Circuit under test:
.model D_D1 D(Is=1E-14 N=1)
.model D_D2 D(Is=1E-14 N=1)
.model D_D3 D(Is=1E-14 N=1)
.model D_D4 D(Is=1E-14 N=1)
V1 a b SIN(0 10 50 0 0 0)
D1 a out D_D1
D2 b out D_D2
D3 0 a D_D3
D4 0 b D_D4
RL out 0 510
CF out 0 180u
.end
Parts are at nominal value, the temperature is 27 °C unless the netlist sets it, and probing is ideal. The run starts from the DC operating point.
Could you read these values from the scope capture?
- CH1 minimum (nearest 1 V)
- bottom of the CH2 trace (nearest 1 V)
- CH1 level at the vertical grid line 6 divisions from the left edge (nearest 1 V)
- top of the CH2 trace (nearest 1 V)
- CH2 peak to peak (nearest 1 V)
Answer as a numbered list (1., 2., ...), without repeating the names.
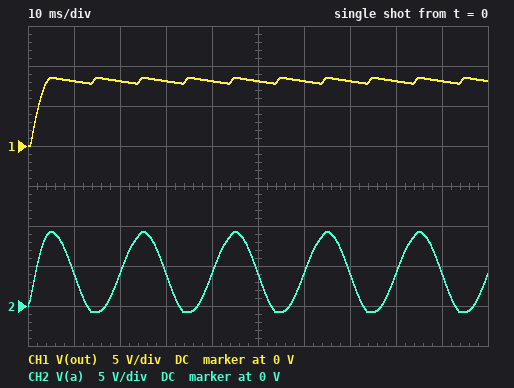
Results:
1. 0 V
2. -1 V
3. 8 V
4. 9 V
5. 10 V
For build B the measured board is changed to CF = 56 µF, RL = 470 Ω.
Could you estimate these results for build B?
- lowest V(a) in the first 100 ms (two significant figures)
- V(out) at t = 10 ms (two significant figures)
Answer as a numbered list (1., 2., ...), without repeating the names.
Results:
1. -780 mV
2. 7.2 V
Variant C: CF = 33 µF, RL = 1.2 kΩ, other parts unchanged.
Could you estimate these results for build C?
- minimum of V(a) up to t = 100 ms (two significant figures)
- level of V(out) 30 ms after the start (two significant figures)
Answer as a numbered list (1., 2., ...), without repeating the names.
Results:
1. -760 mV
2. 7.6 V
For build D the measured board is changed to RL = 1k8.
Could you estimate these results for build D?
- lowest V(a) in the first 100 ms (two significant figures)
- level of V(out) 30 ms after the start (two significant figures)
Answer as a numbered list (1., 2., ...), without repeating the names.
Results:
1. -770 mV
2. 8.4 V
